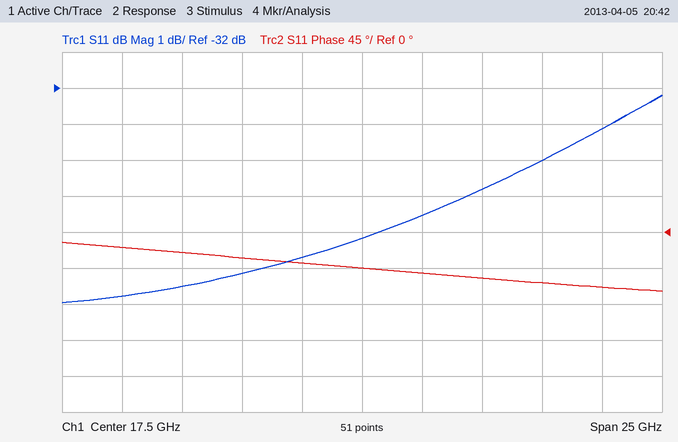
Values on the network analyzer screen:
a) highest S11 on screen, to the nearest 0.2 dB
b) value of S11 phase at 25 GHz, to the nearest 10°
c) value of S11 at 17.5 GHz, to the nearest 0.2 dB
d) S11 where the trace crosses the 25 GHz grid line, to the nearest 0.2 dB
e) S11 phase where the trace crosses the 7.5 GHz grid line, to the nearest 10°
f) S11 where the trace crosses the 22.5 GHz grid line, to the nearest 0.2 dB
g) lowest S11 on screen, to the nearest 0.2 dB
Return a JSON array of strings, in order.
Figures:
["-32.2 dB", "-60°", "-36.2 dB", "-34.0 dB", "-20°", "-34.8 dB", "-38.0 dB"]
